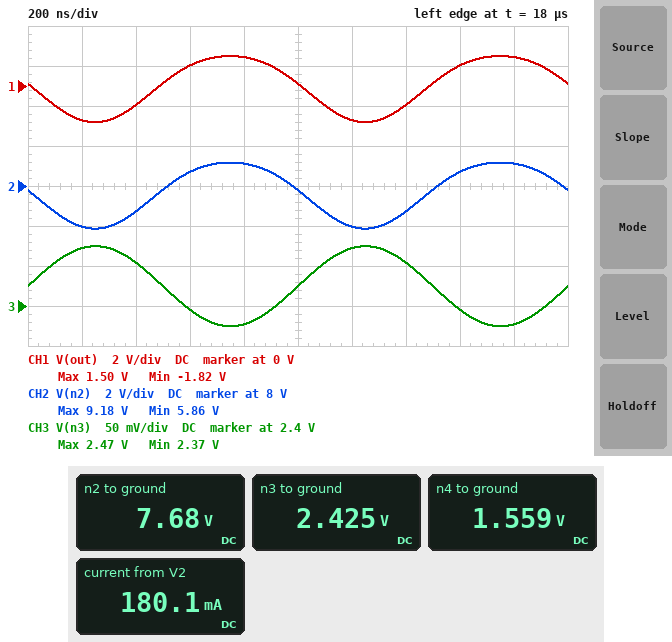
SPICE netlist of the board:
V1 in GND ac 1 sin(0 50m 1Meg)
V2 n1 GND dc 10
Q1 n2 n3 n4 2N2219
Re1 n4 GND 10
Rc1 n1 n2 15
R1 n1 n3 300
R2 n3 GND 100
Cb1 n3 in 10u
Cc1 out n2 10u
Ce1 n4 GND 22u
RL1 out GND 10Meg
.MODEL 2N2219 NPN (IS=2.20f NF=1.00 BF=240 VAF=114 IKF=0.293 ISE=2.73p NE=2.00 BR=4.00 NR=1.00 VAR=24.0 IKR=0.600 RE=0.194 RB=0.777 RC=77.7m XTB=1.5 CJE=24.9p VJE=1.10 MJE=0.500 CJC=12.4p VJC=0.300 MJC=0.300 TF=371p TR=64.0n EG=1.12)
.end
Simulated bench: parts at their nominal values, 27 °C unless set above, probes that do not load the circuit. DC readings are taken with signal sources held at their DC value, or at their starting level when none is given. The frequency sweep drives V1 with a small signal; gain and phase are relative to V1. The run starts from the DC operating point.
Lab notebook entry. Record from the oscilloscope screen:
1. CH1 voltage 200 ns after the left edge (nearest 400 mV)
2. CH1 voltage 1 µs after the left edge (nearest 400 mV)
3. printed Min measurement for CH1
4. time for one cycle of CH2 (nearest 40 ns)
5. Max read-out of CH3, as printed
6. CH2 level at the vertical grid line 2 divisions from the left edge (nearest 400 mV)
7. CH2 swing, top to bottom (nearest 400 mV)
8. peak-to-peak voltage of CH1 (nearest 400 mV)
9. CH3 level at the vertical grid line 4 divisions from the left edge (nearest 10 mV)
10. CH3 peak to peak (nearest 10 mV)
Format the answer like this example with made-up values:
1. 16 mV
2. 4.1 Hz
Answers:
1. -1.6 V
2. 0 V
3. -1.82 V
4. 1.00 µs
5. 2.47 V
6. 6.8 V
7. 3.2 V
8. 3.2 V
9. 2.38 V
10. 100 mV
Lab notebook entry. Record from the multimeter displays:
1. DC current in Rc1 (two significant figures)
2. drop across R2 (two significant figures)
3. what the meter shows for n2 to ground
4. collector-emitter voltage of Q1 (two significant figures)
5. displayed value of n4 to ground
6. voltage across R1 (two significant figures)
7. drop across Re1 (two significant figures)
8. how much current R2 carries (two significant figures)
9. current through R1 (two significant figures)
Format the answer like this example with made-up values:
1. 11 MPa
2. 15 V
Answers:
1. 150 mA
2. 2.4 V
3. 7.68 V
4. 6.1 V
5. 1.559 V
6. 7.6 V
7. 1.6 V
8. 24 mA
9. 25 mA
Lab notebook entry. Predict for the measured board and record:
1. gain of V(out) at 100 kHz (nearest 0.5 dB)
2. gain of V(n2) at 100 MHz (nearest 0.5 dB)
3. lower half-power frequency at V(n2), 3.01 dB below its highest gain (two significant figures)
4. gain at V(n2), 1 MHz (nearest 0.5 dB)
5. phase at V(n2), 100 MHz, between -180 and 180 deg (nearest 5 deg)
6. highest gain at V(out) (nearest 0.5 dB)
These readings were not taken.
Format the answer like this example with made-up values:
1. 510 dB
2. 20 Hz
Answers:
1. 30.5 dB
2. 29.5 dB
3. 18 kHz
4. 31.0 dB
5. 145 deg
6. 31.0 dB
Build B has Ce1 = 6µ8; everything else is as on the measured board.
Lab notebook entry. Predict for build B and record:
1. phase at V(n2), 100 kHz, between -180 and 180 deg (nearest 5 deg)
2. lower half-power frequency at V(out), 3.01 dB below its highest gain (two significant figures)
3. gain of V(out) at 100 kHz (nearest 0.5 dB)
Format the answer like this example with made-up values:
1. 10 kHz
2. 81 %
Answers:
1. -150 deg
2. 57 kHz
3. 29.5 dB
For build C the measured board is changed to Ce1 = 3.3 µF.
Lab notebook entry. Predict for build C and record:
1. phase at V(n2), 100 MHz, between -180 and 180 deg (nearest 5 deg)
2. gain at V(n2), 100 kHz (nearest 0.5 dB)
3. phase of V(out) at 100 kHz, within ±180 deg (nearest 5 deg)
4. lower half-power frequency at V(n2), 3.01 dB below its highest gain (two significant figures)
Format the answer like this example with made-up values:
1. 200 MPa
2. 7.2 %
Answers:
1. 145 deg
2. 27.0 dB
3. -135 deg
4. 120 kHz
